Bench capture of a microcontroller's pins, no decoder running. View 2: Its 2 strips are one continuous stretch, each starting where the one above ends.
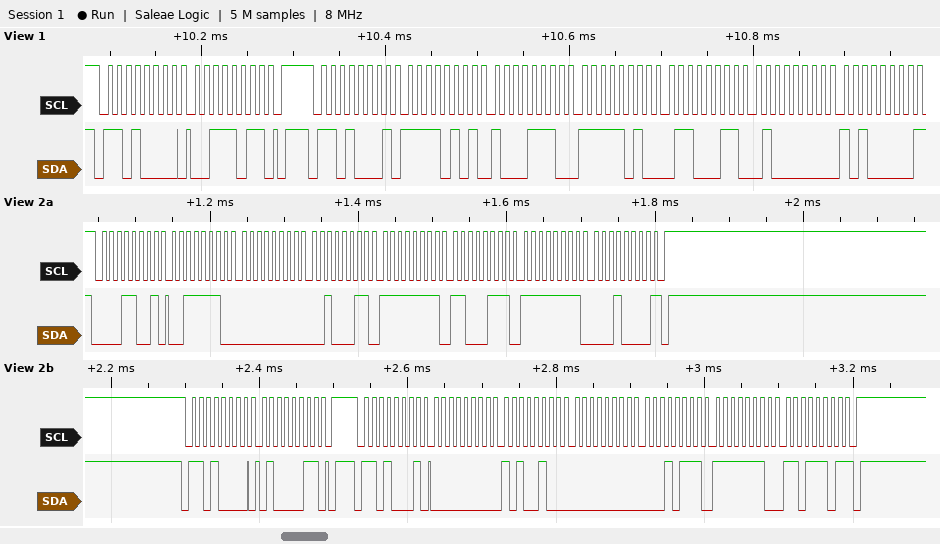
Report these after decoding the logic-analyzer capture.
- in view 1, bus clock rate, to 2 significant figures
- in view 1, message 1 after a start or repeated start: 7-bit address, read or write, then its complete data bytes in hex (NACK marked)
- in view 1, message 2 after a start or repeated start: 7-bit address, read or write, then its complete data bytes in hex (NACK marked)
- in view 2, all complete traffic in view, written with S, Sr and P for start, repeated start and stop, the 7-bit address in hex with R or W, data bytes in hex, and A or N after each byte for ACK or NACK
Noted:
100 kHz
0x68 write: 3B
0x68 read: F5 8E FA 63 40 A0 NACK
S 0CR A 3E A 00 A 23 A FF A C7 A FF A 10 N P S 68W A 43 A P S 68R A 00 A A4 A 00 A 17 A FE A DD N P
